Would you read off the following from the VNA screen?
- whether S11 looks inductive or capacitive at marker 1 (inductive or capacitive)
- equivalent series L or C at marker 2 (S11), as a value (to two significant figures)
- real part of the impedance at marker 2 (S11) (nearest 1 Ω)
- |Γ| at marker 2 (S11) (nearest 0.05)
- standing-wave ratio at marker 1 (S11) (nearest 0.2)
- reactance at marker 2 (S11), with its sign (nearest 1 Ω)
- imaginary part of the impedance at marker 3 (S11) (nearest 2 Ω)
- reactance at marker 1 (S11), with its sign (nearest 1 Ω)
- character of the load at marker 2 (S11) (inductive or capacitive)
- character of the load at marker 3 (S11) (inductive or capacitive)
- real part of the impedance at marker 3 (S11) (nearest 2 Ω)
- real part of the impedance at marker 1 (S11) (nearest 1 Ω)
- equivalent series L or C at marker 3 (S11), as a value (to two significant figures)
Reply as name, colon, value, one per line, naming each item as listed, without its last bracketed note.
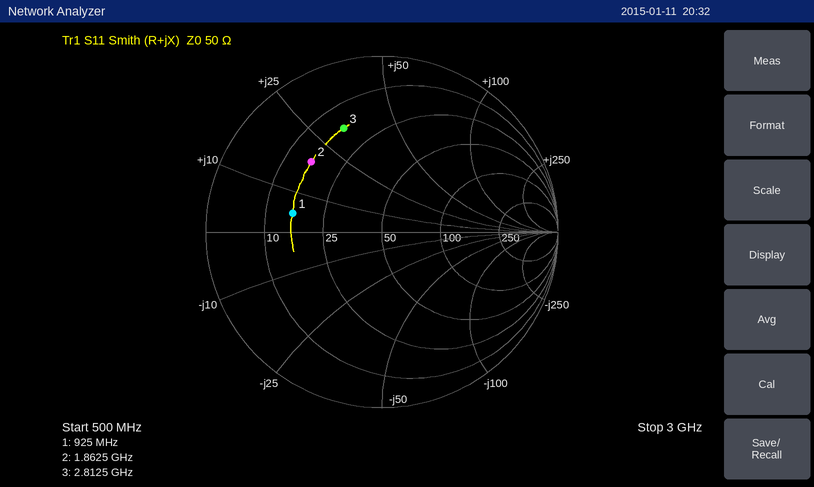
whether S11 looks inductive or capacitive at marker 1: inductive
equivalent series L or C at marker 2 (S11), as a value: 1.6 nH
real part of the impedance at marker 2 (S11): 16 Ω
|Γ| at marker 2 (S11): 0.55
standing-wave ratio at marker 1 (S11): 3.2
reactance at marker 2 (S11), with its sign: +19 Ω
imaginary part of the impedance at marker 3 (S11): +32 Ω
reactance at marker 1 (S11), with its sign: +5 Ω
character of the load at marker 2 (S11): inductive
character of the load at marker 3 (S11): inductive
real part of the impedance at marker 3 (S11): 16 Ω
real part of the impedance at marker 1 (S11): 16 Ω
equivalent series L or C at marker 3 (S11), as a value: 1.8 nH
